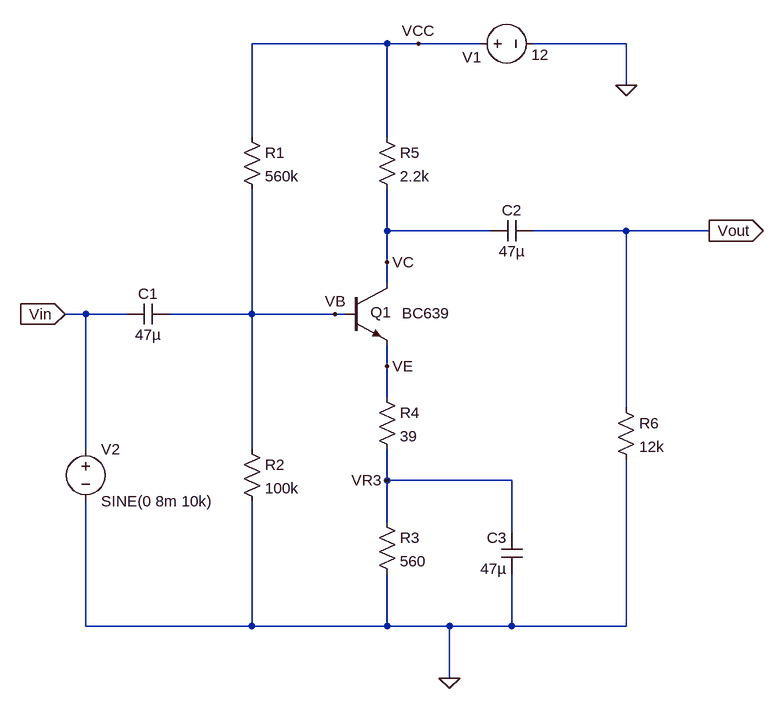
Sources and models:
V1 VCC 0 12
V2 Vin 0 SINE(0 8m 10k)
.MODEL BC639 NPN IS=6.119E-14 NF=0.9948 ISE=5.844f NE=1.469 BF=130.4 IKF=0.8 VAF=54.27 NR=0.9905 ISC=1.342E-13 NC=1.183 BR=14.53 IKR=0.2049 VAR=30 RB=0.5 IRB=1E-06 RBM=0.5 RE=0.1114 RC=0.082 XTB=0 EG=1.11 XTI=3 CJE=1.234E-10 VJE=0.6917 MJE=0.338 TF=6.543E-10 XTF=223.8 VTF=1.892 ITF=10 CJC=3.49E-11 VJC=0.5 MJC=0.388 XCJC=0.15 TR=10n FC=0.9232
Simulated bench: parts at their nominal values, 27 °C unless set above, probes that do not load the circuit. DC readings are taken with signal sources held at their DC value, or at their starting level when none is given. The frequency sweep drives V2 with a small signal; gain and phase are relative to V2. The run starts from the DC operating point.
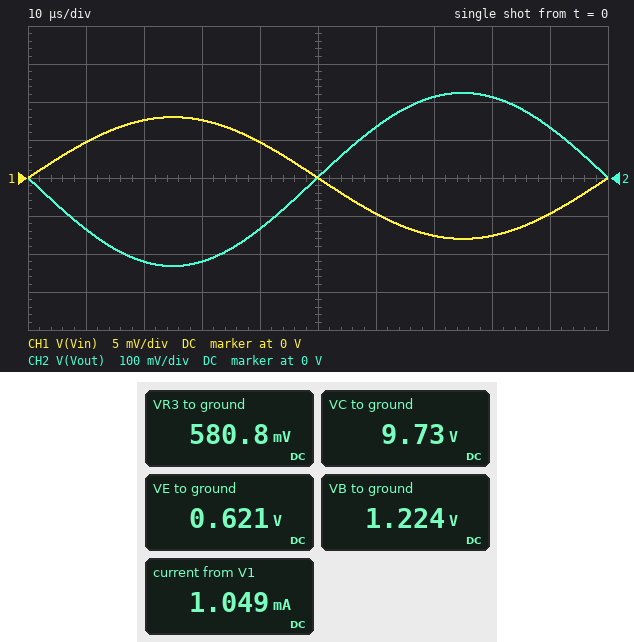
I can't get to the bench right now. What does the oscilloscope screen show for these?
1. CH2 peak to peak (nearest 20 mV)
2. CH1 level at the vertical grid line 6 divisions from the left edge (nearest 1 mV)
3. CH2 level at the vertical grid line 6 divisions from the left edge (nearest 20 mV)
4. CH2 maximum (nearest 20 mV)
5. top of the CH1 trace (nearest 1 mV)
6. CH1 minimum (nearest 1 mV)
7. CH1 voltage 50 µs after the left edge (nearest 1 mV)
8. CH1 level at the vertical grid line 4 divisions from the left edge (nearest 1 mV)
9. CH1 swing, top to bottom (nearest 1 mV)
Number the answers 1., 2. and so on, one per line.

1. 460 mV
2. -5 mV
3. 140 mV
4. 220 mV
5. 8 mV
6. -8 mV
7. 0 V
8. 5 mV
9. 16 mV
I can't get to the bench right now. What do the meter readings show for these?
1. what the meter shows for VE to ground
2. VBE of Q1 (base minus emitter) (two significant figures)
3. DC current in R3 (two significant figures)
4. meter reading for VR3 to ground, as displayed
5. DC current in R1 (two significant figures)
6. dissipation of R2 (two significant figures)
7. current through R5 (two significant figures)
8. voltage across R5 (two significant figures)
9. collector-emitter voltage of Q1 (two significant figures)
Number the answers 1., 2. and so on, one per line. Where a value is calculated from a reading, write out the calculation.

1. 0.621 V
2. 1.224 V - 621 mV = 600 mV
3. (580.8 mV) / 560 Ω = 1.0 mA
4. 580.8 mV
5. (12 V - 1.224 V) / 560 kΩ = 19 µA
6. (1.224 V)^2 / 100 kΩ = 15 µW
7. (12 V - 9.73 V) / 2.2 kΩ = 1.0 mA
8. 12 V - 9.73 V = 2.3 V
9. 9.73 V - 621 mV = 9.1 V
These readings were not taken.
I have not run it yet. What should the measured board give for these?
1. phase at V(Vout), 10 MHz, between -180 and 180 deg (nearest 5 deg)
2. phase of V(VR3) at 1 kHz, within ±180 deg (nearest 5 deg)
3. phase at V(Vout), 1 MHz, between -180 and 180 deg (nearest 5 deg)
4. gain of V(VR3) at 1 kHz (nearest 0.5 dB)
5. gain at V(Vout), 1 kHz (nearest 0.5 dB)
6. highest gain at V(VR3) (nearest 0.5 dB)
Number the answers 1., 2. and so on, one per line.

1. 110 deg
2. -85 deg
3. 170 deg
4. -25.5 dB
5. 29.0 dB
6. -1.0 dB
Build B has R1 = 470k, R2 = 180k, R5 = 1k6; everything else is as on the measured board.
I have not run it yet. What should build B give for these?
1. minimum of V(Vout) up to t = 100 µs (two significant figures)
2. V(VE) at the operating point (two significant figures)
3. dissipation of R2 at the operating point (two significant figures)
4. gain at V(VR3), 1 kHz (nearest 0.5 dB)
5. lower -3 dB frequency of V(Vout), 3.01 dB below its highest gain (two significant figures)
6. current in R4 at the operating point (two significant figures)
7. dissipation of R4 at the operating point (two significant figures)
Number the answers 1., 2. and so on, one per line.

1. -210 mV
2. 1.1 V
3. 16 µW
4. -24.0 dB
5. 69 Hz
6. 1.8 mA
7. 130 µW
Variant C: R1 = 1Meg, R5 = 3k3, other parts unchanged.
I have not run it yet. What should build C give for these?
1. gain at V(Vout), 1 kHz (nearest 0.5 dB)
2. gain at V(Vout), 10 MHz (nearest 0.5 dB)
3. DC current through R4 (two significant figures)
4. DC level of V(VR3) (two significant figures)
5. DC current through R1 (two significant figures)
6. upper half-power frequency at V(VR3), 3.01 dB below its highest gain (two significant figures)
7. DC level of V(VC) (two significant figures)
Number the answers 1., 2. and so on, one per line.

1. 28.0 dB
2. 22.0 dB
3. 430 µA
4. 240 mV
5. 11 µA
6. 40 Hz
7. 11 V
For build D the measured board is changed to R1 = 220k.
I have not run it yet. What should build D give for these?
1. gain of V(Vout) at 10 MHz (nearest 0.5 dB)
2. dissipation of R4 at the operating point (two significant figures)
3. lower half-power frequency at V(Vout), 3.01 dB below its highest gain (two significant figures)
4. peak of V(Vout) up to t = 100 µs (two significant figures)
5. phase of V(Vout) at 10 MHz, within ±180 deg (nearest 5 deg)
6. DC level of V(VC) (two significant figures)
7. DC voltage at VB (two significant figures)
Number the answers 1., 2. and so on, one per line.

1. 25.0 dB
2. 310 µW
3. 75 Hz
4. 300 mV
5. 105 deg
6. 5.8 V
7. 2.3 V
